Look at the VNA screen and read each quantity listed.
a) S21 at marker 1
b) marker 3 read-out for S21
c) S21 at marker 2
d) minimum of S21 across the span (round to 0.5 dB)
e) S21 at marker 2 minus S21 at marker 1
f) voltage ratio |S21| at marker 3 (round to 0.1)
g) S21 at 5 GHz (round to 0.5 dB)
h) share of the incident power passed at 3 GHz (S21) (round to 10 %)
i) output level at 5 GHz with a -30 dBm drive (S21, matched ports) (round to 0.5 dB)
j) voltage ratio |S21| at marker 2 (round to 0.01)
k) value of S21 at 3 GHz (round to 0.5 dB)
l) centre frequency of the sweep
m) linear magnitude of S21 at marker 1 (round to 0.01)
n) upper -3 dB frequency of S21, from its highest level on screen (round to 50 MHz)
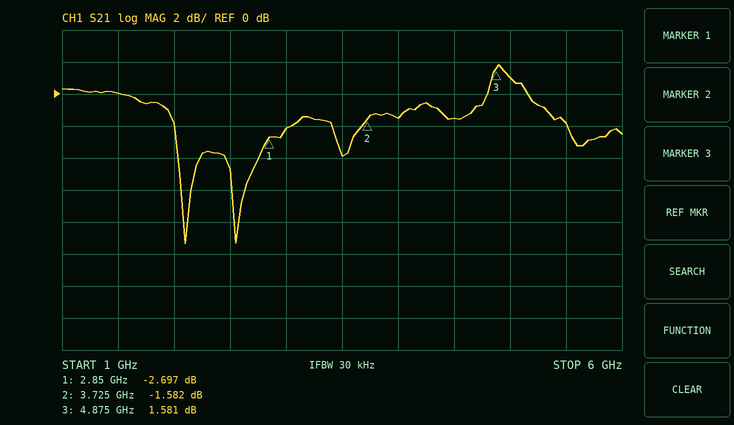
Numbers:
-2.697 dB
1.581 dB
-1.582 dB
-9.5 dB
1.115 dB
1.2
1.0 dB
60 %
-29.0 dBm
0.83
-2.0 dB
3.5 GHz
0.73
5.35 GHz
